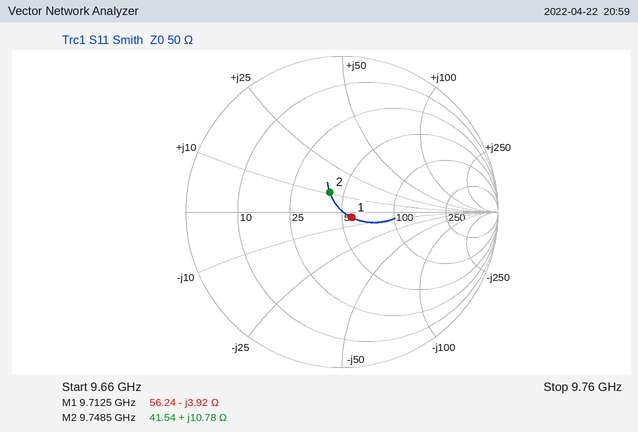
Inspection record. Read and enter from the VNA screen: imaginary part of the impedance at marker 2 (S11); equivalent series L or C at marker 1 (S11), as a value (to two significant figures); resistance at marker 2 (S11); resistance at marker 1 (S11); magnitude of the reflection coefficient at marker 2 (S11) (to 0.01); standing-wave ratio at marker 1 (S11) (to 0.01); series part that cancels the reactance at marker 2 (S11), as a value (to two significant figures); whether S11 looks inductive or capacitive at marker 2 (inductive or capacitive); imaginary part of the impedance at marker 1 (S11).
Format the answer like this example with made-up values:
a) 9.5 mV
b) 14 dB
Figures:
a) +10.78 Ω
b) 4.2 pF
c) 41.54 Ω
d) 56.24 Ω
e) 0.15
f) 1.15
g) 1.5 pF
h) inductive
i) -3.92 Ω
